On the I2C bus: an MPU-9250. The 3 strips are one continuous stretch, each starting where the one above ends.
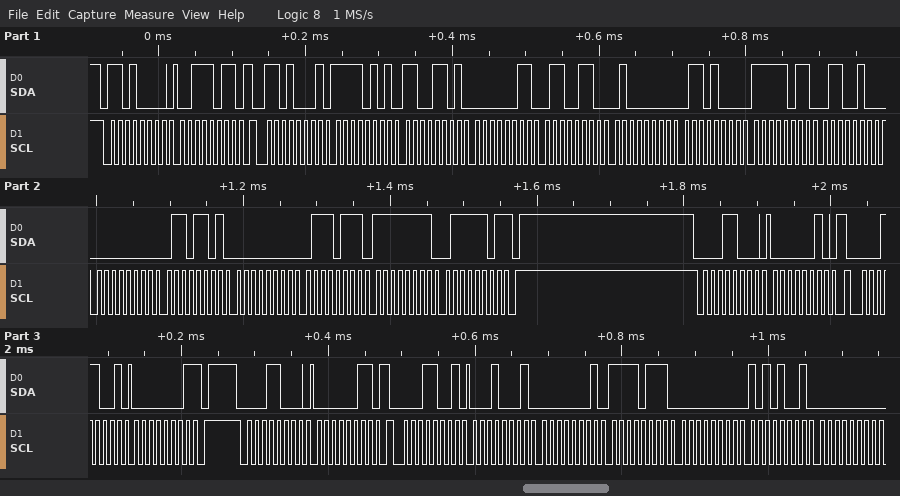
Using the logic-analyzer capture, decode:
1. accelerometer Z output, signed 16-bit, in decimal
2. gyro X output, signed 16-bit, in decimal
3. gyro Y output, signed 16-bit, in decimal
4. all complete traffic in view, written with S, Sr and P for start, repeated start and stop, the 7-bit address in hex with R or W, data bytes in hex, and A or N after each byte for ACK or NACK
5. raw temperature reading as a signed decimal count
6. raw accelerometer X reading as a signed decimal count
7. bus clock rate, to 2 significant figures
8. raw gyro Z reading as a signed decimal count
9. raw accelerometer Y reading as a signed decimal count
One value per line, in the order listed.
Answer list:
16488
109
119
S 68W A 3B A Sr 68R A F5 A CD A 03 A 66 A 40 A 68 A FB A 64 A 00 A 6D A 00 A 77 A FF A 7D N P S 0CW A 02 A Sr 0CR A 01 N P S 0CW A 03 A Sr 0CR A 11 A 01 A F7 A 00 A A9 A 00 A
-1180
-2611
100 kHz
-131
870
